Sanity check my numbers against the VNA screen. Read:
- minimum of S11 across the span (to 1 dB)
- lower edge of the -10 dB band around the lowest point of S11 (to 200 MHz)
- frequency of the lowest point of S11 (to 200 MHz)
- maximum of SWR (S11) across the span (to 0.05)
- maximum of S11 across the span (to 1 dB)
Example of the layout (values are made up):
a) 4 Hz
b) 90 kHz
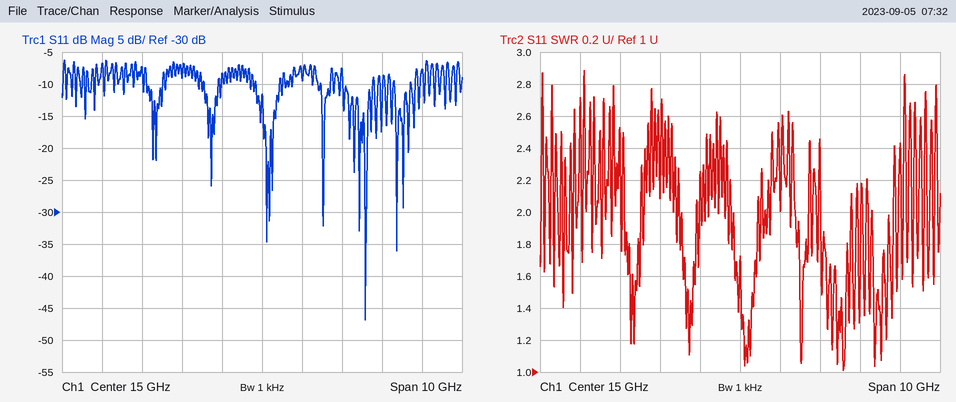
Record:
a) -47 dB
b) 17.0 GHz
c) 17.6 GHz
d) 2.90
e) -6 dB
